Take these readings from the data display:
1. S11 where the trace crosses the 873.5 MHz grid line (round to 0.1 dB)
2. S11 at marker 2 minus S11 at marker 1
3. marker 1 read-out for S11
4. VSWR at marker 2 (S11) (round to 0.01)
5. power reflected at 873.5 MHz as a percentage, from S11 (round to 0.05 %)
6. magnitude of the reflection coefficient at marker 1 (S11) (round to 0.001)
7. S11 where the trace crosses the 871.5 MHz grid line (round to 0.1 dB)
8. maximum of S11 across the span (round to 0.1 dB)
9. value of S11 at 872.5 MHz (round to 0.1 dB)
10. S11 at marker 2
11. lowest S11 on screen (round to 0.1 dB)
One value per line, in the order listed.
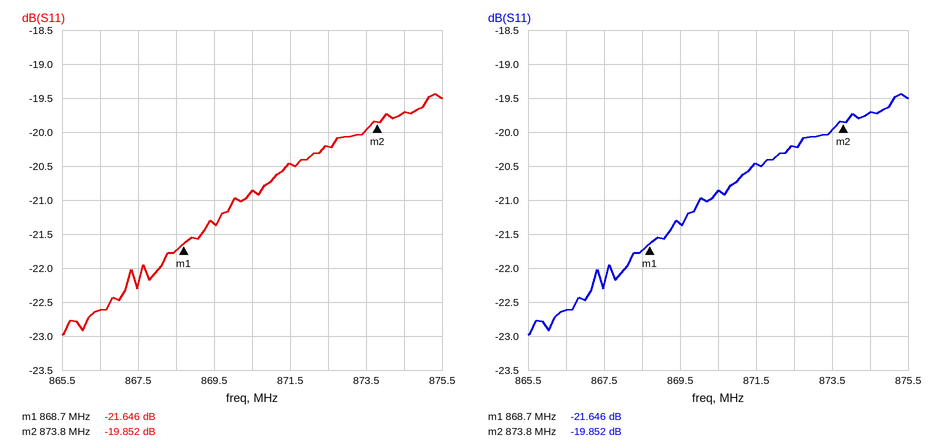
-20.0 dB
1.794 dB
-21.646 dB
1.23
1.00 %
0.083
-20.5 dB
-19.4 dB
-20.2 dB
-19.852 dB
-23.0 dB
